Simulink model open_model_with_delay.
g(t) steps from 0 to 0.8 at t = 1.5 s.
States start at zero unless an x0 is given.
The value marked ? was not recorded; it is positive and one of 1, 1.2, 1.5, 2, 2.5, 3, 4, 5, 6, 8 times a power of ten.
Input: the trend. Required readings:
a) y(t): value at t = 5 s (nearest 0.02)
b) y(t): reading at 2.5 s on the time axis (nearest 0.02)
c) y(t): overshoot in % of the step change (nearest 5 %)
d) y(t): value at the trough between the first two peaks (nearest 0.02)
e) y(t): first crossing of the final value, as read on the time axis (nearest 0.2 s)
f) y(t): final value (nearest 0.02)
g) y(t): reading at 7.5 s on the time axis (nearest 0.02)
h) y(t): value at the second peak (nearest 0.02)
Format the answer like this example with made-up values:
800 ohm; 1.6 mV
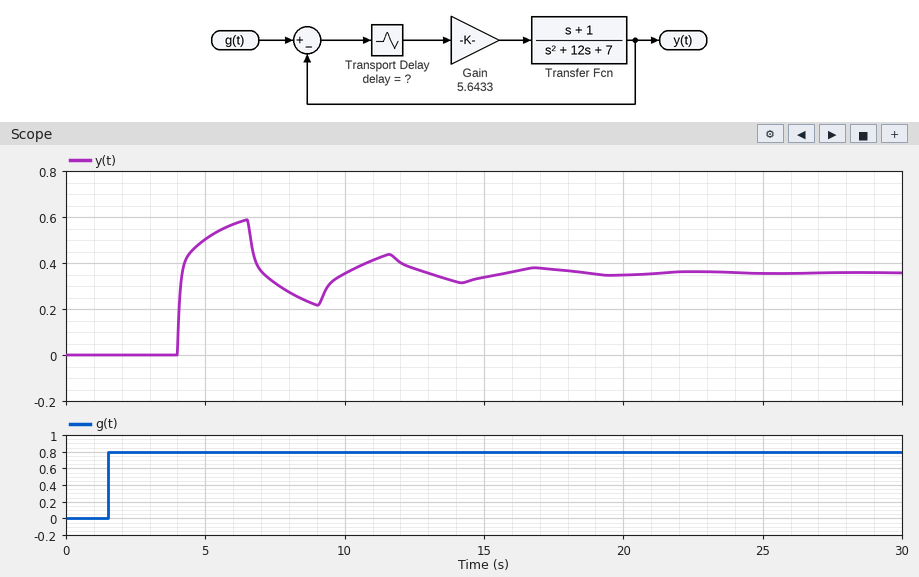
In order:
0.50; 0.00; 65 %; 0.22; 4.2 s; 0.36; 0.32; 0.44
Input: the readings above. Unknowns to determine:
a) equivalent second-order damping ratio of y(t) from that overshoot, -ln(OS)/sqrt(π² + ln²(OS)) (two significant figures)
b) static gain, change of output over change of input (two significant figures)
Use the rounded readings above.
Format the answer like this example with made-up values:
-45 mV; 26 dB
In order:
0.14; 0.45
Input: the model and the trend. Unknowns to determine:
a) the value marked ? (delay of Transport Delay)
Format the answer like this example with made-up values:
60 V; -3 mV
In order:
2.5
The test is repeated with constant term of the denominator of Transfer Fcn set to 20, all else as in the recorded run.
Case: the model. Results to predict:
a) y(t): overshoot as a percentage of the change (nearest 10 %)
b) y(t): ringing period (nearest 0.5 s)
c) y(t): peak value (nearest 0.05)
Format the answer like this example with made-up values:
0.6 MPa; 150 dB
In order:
100 %; 5.0 s; 0.35
